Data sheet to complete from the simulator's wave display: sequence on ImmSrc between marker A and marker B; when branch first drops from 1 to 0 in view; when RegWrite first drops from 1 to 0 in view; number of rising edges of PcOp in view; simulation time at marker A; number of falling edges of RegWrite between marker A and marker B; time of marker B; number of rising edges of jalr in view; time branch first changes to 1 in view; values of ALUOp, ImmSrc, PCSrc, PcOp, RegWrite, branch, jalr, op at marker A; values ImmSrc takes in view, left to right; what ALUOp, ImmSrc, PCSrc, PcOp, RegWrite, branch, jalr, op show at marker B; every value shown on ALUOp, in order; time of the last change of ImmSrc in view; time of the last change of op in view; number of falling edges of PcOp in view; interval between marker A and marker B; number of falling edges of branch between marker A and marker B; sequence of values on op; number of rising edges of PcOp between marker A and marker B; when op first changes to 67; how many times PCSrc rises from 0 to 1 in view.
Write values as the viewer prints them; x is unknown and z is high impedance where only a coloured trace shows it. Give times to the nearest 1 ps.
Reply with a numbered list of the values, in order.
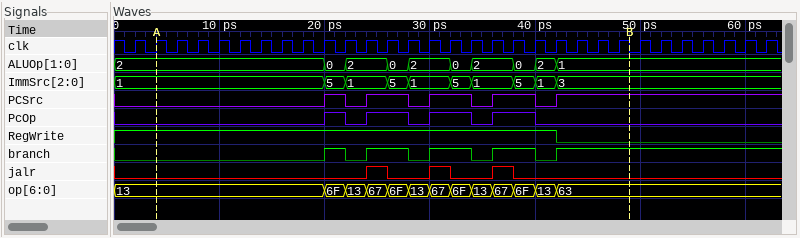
1. 1, 5, 1, 5, 1, 5, 1, 5, 1, 3
2. 22 ps
3. 42 ps
4. 4
5. 4 ps
6. 1
7. 49 ps
8. 3
9. 20 ps
10. ALUOp=2, ImmSrc=1, PCSrc=0, PcOp=0, RegWrite=1, branch=0, jalr=0, op=13
11. 1, 5, 1, 5, 1, 5, 1, 5, 1, 3
12. ALUOp=1, ImmSrc=3, PCSrc=1, PcOp=0, RegWrite=0, branch=1, jalr=0, op=63
13. 2, 0, 2, 0, 2, 0, 2, 0, 2, 1
14. 42 ps
15. 42 ps
16. 4
17. 45 ps
18. 4
19. 13, 6F, 13, 67, 6F, 13, 67, 6F, 13, 67, 6F, 13, 63
20. 4
21. 24 ps
22. 5
